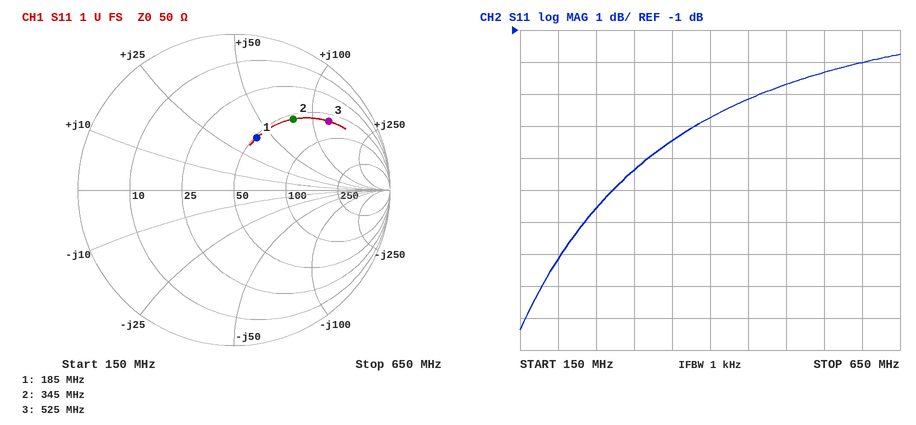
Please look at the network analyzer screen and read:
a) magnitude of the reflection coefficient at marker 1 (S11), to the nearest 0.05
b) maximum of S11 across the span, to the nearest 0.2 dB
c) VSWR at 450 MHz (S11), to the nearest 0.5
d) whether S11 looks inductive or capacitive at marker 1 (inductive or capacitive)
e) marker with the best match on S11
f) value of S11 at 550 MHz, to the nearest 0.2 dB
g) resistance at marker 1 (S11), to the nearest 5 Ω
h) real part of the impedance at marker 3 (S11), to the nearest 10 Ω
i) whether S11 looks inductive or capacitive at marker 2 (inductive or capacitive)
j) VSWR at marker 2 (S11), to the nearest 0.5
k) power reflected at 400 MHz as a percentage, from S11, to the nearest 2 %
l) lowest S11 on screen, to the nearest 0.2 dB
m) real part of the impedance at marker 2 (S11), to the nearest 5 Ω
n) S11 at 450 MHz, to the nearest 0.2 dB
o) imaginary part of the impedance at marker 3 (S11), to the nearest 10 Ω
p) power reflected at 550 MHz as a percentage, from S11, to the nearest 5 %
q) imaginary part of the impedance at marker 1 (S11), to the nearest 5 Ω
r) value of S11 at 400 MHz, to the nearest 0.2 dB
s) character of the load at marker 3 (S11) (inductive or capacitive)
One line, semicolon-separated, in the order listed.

0.35; -1.8 dB; 5.5; inductive; marker 1; -2.4 dB; 50 Ω; 60 Ω; inductive; 4.0; 42 %; -10.4 dB; 55 Ω; -3.2 dB; +130 Ω; 60 %; +40 Ω; -3.8 dB; inductive
